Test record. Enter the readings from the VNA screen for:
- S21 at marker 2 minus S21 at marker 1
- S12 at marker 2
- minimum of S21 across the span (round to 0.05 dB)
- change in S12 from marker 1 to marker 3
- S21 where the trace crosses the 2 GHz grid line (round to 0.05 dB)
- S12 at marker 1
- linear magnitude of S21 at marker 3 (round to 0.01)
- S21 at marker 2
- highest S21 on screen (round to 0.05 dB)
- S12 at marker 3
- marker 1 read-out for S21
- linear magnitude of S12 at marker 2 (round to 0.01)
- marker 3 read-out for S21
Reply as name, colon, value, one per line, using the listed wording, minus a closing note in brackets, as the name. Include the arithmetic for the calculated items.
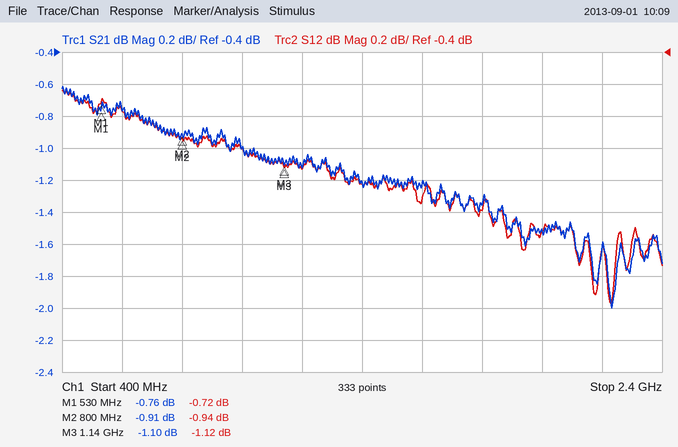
S21 at marker 2 minus S21 at marker 1: -0.91 − (-0.76) = -0.15 dB
S12 at marker 2: -0.94 dB
minimum of S21 across the span: -2.00 dB
change in S12 from marker 1 to marker 3: -1.12 − (-0.72) = -0.40 dB
S21 where the trace crosses the 2 GHz grid line: -1.50 dB
S12 at marker 1: -0.72 dB
linear magnitude of S21 at marker 3: 10^(-1.1/20) ≈ 0.88
S21 at marker 2: -0.91 dB
highest S21 on screen: -0.60 dB
S12 at marker 3: -1.12 dB
marker 1 read-out for S21: -0.76 dB
linear magnitude of S12 at marker 2: 10^(-0.94/20) ≈ 0.90
marker 3 read-out for S21: -1.10 dB
